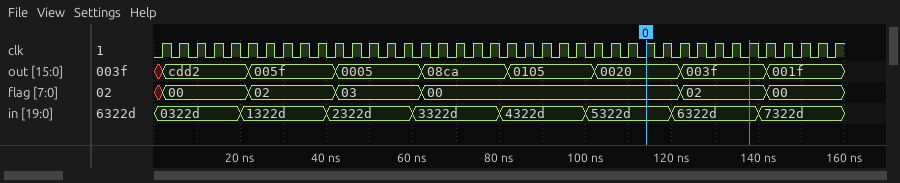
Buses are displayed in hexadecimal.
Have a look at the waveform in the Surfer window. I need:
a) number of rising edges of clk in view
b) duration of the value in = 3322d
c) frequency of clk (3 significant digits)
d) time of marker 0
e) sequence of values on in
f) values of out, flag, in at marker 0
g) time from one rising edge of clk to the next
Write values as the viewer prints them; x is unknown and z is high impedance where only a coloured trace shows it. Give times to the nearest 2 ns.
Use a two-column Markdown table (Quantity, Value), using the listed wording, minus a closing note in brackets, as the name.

| Quantity | Value |
|---|---|
| number of rising edges of clk in view | 40 |
| duration of the value in = 3322d | 20 ns |
| frequency of clk | 250 MHz |
| time of marker 0 | 114 ns |
| sequence of values on in | 0322d, 1322d, 2322d, 3322d, 4322d, 5322d, 6322d, 7322d |
| values of out, flag, in at marker 0 | out=0020, flag=00, in=5322d |
| time from one rising edge of clk to the next | 4 ns |
